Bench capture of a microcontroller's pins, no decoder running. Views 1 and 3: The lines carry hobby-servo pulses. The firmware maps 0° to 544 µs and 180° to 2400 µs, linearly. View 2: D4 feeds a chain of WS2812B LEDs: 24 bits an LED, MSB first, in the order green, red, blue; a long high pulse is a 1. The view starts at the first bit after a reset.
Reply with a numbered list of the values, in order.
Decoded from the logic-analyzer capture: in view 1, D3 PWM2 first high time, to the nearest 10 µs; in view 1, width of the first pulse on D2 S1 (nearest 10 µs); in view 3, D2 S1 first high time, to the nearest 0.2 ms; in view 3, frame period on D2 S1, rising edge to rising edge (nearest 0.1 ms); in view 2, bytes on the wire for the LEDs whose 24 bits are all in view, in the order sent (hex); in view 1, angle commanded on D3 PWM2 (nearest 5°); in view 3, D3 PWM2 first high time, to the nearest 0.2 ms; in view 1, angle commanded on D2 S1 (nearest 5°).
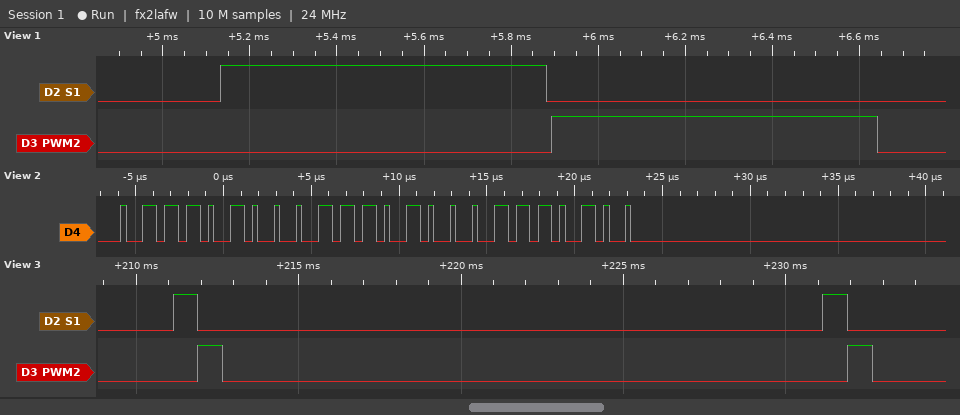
1. 750 µs
2. 750 µs
3. 0.8 ms
4. 20.0 ms
5. 74 74 74
6. 20°
7. 0.8 ms
8. 20°
